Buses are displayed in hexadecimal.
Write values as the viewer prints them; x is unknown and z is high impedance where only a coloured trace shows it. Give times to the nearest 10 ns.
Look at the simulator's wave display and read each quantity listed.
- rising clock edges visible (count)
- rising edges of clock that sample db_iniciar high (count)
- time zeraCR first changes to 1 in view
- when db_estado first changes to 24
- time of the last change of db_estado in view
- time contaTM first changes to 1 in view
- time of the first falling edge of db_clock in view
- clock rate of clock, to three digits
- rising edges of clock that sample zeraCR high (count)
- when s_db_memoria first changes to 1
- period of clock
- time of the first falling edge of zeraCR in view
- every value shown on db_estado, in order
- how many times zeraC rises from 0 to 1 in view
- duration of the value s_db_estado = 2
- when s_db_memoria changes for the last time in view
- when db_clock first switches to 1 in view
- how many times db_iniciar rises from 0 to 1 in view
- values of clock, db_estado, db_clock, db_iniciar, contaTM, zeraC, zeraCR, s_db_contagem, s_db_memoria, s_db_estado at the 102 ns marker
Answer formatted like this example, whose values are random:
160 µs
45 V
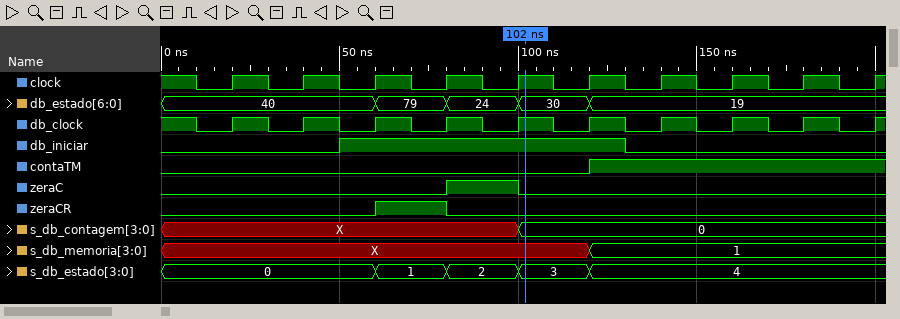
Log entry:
10
4
60 ns
80 ns
120 ns
120 ns
10 ns
50.0 MHz
1
120 ns
20 ns
80 ns
40, 79, 24, 30, 19
1
20 ns
120 ns
20 ns
1
clock=1, db_estado=30, db_clock=1, db_iniciar=1, contaTM=0, zeraC=0, zeraCR=0, s_db_contagem=0, s_db_memoria=X, s_db_estado=3
